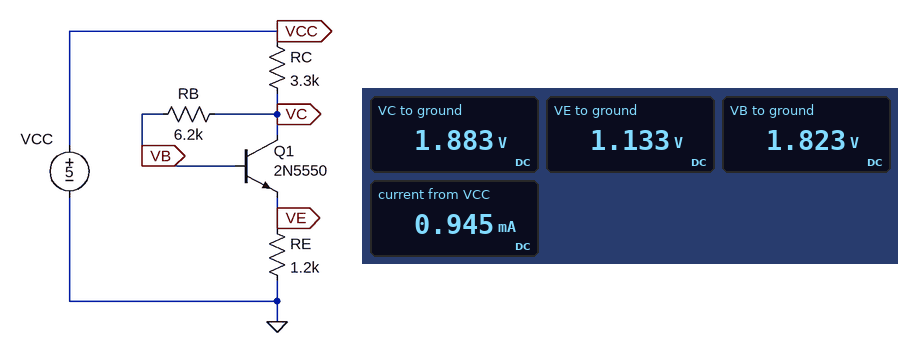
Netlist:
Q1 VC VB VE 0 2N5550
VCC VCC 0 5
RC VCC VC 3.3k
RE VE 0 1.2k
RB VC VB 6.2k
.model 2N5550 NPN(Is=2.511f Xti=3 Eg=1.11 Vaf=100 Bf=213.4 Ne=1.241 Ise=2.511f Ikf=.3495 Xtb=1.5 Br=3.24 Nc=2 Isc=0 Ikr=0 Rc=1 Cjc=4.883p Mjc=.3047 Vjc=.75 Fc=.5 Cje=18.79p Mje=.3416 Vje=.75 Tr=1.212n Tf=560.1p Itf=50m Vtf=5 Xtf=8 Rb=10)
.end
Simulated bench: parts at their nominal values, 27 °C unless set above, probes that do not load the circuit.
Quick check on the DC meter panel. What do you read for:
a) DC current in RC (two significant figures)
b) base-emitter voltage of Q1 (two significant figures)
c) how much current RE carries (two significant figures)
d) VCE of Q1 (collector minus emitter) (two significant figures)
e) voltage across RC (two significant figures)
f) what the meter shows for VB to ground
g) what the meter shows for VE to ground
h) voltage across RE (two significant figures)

940 µA
690 mV
940 µA
750 mV
3.1 V
1.823 V
1.133 V
1.1 V
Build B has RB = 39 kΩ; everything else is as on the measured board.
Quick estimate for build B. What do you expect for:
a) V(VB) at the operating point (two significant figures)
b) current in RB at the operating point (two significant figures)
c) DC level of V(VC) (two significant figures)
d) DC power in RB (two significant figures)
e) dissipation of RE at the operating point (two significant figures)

1.7 V
9.1 µA
2.1 V
3.2 µW
930 µW
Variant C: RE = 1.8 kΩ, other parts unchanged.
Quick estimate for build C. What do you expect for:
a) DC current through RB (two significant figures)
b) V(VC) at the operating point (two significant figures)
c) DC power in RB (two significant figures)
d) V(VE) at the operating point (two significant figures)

8.7 µA
2.2 V
470 nW
1.5 V
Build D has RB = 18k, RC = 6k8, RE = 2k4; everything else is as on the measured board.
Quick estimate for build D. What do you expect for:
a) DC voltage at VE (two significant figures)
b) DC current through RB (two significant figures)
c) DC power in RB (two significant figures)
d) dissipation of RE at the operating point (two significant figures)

1.1 V
5.1 µA
470 nW
510 µW
